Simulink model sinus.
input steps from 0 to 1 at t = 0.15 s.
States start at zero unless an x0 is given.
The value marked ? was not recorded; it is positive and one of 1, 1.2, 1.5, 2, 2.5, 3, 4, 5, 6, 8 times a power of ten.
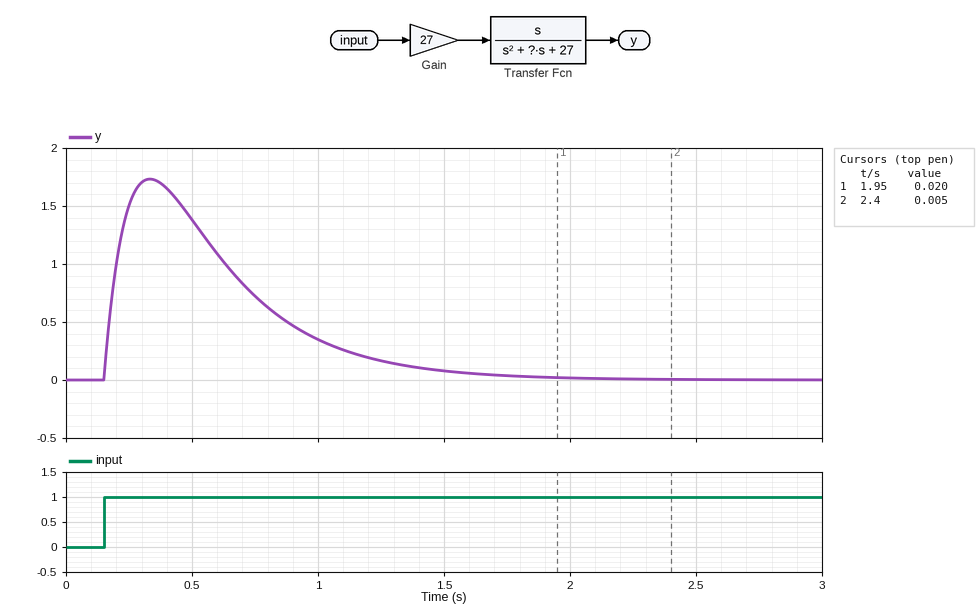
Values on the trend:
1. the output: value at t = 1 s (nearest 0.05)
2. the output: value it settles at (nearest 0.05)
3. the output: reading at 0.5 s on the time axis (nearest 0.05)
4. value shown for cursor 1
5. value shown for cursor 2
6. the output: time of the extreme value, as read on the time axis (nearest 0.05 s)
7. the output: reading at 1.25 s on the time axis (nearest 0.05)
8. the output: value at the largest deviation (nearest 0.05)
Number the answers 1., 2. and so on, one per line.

1. 0.35
2. 0.00
3. 1.40
4. 0.020
5. 0.005
6. 0.35 s
7. 0.15
8. 1.75
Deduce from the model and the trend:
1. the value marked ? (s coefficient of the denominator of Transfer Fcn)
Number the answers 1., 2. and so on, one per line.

1. 12
